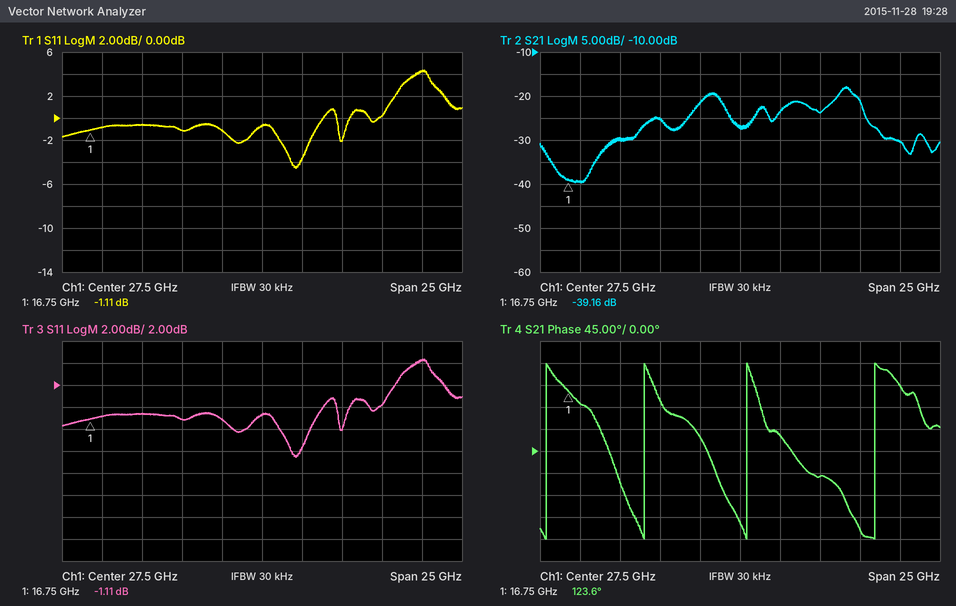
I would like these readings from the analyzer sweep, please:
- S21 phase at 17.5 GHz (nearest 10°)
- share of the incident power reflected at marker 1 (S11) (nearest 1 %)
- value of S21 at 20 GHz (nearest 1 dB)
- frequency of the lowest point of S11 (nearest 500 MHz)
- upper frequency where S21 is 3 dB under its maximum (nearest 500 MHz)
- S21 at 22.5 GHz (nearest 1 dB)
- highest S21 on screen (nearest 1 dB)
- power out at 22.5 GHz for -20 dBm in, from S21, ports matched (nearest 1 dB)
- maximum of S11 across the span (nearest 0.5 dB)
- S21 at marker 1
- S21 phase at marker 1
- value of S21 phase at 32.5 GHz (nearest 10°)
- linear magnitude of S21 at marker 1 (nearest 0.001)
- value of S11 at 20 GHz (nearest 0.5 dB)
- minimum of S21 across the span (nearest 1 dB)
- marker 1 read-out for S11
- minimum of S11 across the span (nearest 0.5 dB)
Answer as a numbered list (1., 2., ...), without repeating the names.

1. 100°
2. 77 %
3. -30 dB
4. 29.5 GHz
5. 35.0 GHz
6. -25 dB
7. -18 dB
8. -45 dBm
9. 4.5 dB
10. -39.16 dB
11. 123.6°
12. -50°
13. 0.011
14. -0.5 dB
15. -40 dB
16. -1.11 dB
17. -4.5 dB
